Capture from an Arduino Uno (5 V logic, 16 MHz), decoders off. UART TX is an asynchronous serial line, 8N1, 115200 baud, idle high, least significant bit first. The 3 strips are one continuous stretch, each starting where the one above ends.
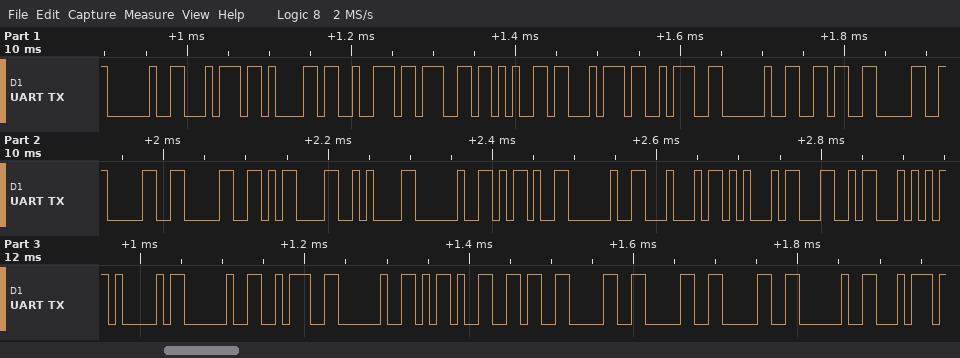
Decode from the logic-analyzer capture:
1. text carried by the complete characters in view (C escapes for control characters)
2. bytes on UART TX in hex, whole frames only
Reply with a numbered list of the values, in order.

1. " target: 6000\r\n - DELTA : -6000 t"
2. 0x20 0x74 0x61 0x72 0x67 0x65 0x74 0x3A 0x20 0x36 0x30 0x30 0x30 0x0D 0x0A 0x20 0x2D 0x20 0x44 0x45 0x4C 0x54 0x41 0x20 0x3A 0x20 0x2D 0x36 0x30 0x30 0x30 0x20 0x74
